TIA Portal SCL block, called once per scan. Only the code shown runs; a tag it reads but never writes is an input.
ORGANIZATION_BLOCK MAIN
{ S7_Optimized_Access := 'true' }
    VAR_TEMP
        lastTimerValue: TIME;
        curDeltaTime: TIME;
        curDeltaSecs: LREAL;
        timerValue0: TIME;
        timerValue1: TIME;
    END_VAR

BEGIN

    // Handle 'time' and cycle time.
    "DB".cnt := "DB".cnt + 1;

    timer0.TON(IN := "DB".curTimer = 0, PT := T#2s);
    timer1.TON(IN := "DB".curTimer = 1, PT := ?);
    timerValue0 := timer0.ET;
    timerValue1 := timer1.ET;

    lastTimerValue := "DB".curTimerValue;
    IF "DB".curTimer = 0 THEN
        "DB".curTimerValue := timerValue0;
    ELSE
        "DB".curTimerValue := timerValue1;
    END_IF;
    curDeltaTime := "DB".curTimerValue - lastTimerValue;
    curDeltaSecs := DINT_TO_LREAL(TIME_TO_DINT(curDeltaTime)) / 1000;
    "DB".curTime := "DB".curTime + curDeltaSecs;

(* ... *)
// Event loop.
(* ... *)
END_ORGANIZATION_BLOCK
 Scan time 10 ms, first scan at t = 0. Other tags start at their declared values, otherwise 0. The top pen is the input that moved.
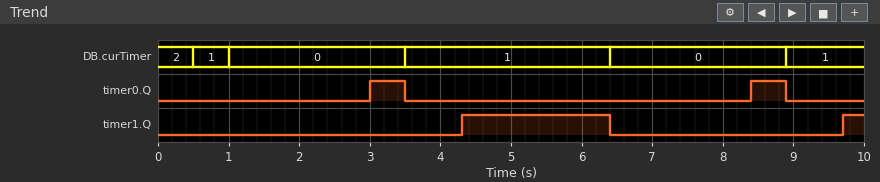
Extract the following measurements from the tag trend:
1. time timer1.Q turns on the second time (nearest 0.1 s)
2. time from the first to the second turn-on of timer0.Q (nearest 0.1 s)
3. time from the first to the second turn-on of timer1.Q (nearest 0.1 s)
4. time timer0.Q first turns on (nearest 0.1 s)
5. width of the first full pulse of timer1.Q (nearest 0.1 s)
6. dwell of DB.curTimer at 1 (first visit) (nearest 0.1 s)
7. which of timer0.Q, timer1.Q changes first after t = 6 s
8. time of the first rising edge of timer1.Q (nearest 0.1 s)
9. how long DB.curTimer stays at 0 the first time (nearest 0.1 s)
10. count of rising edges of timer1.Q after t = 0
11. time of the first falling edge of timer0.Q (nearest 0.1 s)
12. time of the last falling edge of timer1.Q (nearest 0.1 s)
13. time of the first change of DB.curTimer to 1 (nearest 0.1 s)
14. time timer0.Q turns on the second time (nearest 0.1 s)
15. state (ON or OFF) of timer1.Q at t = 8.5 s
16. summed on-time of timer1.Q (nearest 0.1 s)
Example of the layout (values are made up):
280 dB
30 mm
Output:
9.7 s
5.4 s
5.4 s
3.0 s
2.1 s
0.5 s
timer1.Q
4.3 s
2.5 s
2
3.5 s
6.4 s
0.5 s
8.4 s
OFF
2.4 s
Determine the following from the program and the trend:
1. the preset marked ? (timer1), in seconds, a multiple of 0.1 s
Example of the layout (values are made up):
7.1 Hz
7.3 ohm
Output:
0.8 s
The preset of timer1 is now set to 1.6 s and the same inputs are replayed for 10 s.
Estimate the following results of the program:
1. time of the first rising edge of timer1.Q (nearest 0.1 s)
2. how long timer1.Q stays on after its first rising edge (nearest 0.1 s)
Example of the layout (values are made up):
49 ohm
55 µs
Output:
5.1 s
1.3 s
